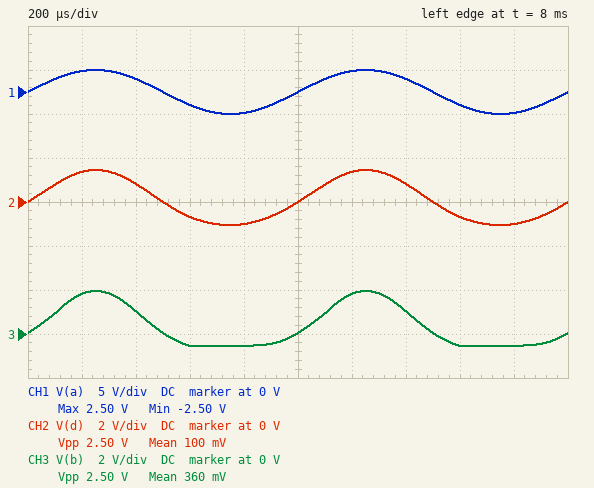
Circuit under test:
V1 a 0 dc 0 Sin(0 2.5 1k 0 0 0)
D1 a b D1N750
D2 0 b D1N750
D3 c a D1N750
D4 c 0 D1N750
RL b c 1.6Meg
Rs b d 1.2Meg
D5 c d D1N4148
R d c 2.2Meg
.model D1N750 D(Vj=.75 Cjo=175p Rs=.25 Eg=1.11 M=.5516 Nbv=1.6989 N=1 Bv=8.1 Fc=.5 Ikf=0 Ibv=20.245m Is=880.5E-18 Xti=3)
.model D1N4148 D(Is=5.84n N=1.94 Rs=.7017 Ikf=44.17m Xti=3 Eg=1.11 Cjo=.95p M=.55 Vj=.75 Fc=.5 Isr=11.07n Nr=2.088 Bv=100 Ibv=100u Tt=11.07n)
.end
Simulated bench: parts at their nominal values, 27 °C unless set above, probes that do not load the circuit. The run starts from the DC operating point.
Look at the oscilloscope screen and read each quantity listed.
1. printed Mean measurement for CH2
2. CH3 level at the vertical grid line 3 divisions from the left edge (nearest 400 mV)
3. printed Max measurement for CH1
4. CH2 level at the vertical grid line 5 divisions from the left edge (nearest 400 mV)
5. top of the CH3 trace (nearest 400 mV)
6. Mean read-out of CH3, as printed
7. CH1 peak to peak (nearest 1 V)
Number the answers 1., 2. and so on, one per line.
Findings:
1. 100 mV
2. -400 mV
3. 2.50 V
4. 0 V
5. 2.0 V
6. 360 mV
7. 5 V
